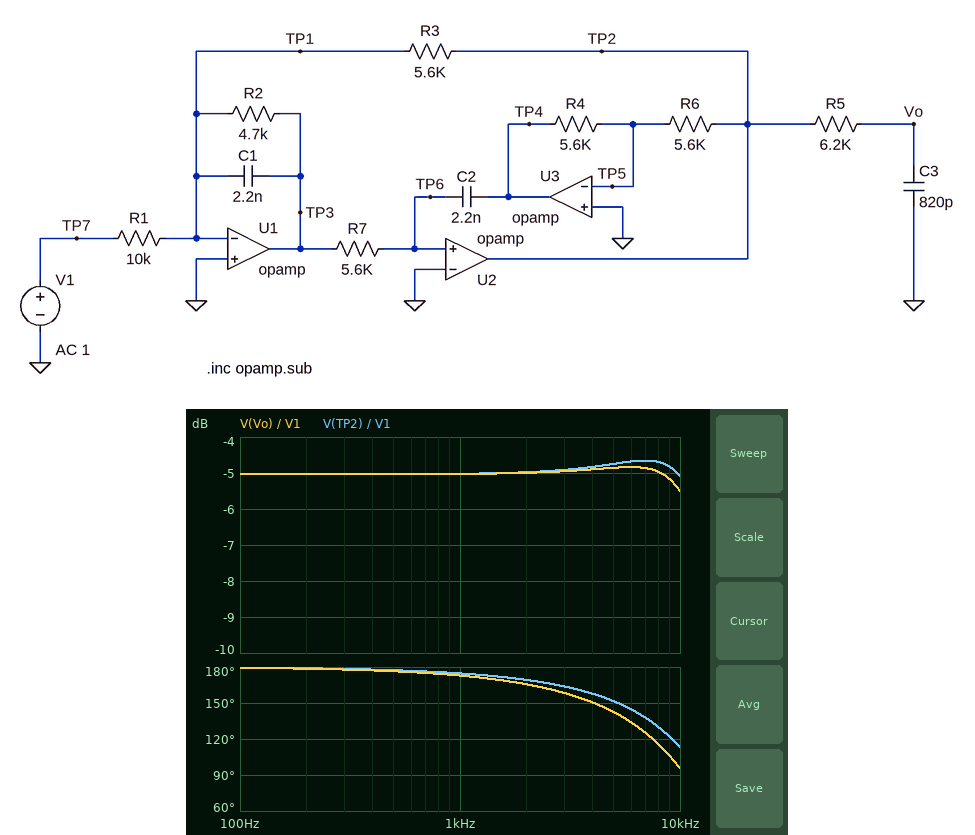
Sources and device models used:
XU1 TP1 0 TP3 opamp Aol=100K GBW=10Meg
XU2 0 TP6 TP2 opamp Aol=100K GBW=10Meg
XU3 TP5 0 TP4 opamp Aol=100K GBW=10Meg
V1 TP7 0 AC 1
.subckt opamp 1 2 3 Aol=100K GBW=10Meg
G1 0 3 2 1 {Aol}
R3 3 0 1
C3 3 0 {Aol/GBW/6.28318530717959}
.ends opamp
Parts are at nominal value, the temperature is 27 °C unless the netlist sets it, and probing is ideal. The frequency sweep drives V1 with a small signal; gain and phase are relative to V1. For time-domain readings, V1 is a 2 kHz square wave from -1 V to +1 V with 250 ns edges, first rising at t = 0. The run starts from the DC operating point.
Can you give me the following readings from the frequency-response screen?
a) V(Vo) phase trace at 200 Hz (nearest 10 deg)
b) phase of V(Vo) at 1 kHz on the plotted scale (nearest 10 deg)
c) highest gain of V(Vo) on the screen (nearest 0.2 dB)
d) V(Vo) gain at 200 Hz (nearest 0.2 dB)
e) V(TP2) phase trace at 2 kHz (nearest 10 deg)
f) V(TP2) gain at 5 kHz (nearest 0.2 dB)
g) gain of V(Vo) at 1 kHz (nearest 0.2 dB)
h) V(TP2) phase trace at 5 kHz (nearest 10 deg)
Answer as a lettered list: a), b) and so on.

a) 180 deg
b) 170 deg
c) -4.8 dB
d) -5.0 dB
e) 170 deg
f) -4.8 dB
g) -5.0 dB
h) 150 deg
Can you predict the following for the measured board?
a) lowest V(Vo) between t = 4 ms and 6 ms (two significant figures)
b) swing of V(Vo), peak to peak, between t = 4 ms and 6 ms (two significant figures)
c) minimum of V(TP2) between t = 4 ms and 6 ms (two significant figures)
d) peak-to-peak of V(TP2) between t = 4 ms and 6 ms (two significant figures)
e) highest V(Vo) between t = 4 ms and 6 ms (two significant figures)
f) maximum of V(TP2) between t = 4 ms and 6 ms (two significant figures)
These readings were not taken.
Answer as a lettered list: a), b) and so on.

a) -660 mV
b) 1.3 V
c) -670 mV
d) 1.3 V
e) 660 mV
f) 670 mV
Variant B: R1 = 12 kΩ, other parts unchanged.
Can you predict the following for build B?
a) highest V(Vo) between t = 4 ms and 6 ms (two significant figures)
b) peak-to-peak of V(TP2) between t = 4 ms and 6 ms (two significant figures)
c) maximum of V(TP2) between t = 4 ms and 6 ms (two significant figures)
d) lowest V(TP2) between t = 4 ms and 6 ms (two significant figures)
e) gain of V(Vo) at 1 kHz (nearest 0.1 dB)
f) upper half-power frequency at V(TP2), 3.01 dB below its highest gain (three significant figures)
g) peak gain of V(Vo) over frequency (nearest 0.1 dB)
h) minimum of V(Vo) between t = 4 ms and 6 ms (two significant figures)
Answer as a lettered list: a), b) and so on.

a) 550 mV
b) 1.1 V
c) 560 mV
d) -560 mV
e) -6.6 dB
f) 14.4 kHz
g) -6.4 dB
h) -550 mV
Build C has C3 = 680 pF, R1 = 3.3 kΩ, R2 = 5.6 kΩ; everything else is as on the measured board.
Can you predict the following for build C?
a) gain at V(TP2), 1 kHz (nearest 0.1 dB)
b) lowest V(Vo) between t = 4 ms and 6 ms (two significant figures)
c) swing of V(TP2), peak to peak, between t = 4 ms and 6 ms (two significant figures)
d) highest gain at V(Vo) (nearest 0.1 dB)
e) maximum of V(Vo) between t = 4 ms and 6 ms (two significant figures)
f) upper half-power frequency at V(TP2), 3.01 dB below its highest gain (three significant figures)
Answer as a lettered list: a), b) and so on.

a) 4.6 dB
b) -2.2 V
c) 4.5 V
d) 5.6 dB
e) 2.2 V
f) 15.1 kHz
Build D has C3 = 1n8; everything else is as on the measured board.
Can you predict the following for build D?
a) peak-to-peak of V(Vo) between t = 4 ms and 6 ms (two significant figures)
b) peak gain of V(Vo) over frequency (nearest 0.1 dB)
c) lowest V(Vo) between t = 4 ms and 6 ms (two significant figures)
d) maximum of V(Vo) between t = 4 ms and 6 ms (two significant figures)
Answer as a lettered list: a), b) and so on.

a) 1.2 V
b) -5.0 dB
c) -620 mV
d) 620 mV
